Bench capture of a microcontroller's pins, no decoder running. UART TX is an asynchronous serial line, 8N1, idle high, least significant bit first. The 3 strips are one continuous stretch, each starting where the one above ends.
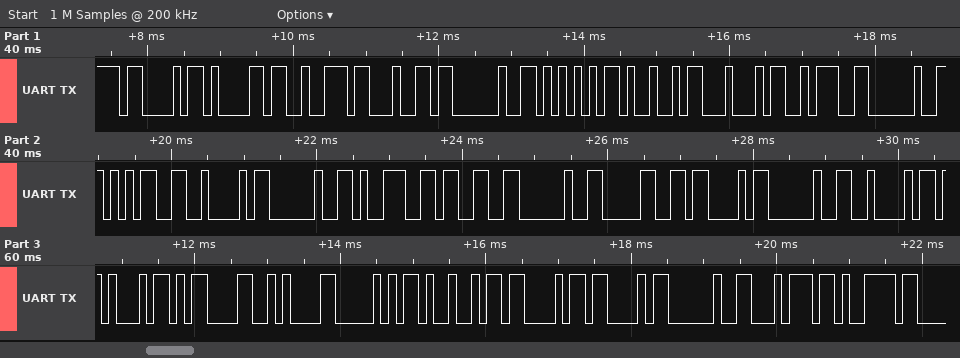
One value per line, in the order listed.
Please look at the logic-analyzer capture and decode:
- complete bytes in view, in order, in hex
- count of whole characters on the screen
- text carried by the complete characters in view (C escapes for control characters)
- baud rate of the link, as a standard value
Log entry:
43 61 72 64 20 55 49 44 3A 20 35 42 20 39 33 20 30 43 20 42 45 0D 0A 50 49 43 43 20 74 79
30
"Card UID: 5B 93 0C BE\r\nPICC ty"
9600 baud
